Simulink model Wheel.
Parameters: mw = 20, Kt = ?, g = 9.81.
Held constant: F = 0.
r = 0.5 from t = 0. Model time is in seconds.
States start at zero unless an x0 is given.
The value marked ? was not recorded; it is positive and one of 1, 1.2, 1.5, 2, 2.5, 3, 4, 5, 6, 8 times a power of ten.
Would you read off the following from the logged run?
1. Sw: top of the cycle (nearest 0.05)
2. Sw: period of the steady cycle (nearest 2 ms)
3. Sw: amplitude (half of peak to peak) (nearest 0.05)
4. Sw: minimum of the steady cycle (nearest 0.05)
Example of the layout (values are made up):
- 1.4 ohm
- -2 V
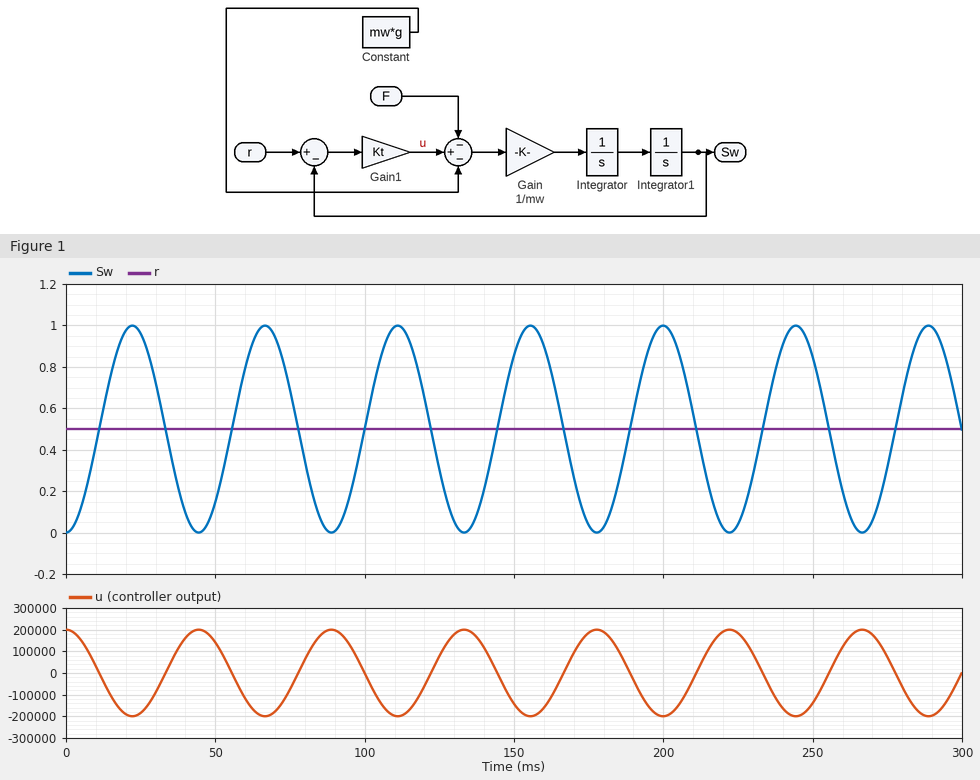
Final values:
- 1.00
- 44 ms
- 0.50
- 0.00
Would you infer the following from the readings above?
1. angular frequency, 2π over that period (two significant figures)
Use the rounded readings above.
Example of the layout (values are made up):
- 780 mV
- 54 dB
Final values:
- 0.14 rad/ms
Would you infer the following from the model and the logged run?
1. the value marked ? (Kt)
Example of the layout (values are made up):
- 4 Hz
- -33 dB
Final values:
- 400000
